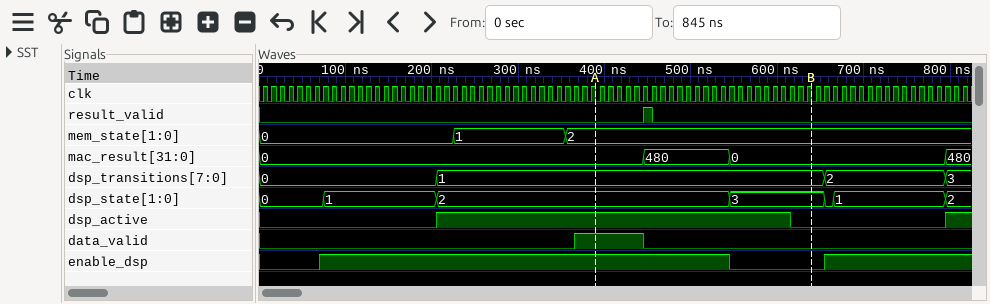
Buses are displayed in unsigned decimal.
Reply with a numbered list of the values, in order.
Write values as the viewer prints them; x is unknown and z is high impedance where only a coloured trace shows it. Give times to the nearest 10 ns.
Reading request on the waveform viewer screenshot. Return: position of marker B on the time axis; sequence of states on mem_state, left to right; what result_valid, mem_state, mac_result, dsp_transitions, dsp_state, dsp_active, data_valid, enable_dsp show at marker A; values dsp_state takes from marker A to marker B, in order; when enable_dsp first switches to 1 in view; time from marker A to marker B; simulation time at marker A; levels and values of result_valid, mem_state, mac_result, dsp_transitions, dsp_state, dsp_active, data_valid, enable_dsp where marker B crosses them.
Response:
1. 640 ns
2. 0, 1, 2
3. result_valid=0, mem_state=2, mac_result=0, dsp_transitions=1, dsp_state=2, dsp_active=1, data_valid=1, enable_dsp=1
4. 2, 3
5. 70 ns
6. 250 ns
7. 390 ns
8. result_valid=0, mem_state=2, mac_result=0, dsp_transitions=1, dsp_state=3, dsp_active=0, data_valid=0, enable_dsp=0
